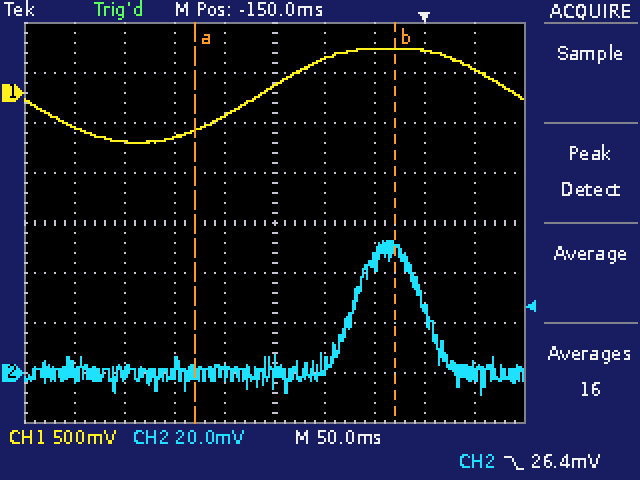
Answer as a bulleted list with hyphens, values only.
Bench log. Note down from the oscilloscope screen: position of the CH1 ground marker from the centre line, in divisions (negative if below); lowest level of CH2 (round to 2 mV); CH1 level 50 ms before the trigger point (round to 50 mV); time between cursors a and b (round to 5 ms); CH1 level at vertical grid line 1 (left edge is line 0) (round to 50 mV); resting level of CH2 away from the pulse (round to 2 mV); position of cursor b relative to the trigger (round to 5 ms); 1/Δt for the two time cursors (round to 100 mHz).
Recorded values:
- +2.6 div
- -8 mV
- 450 mV
- 200 ms
- -350 mV
- 0 mV
- -30 ms
- 5.0 Hz
